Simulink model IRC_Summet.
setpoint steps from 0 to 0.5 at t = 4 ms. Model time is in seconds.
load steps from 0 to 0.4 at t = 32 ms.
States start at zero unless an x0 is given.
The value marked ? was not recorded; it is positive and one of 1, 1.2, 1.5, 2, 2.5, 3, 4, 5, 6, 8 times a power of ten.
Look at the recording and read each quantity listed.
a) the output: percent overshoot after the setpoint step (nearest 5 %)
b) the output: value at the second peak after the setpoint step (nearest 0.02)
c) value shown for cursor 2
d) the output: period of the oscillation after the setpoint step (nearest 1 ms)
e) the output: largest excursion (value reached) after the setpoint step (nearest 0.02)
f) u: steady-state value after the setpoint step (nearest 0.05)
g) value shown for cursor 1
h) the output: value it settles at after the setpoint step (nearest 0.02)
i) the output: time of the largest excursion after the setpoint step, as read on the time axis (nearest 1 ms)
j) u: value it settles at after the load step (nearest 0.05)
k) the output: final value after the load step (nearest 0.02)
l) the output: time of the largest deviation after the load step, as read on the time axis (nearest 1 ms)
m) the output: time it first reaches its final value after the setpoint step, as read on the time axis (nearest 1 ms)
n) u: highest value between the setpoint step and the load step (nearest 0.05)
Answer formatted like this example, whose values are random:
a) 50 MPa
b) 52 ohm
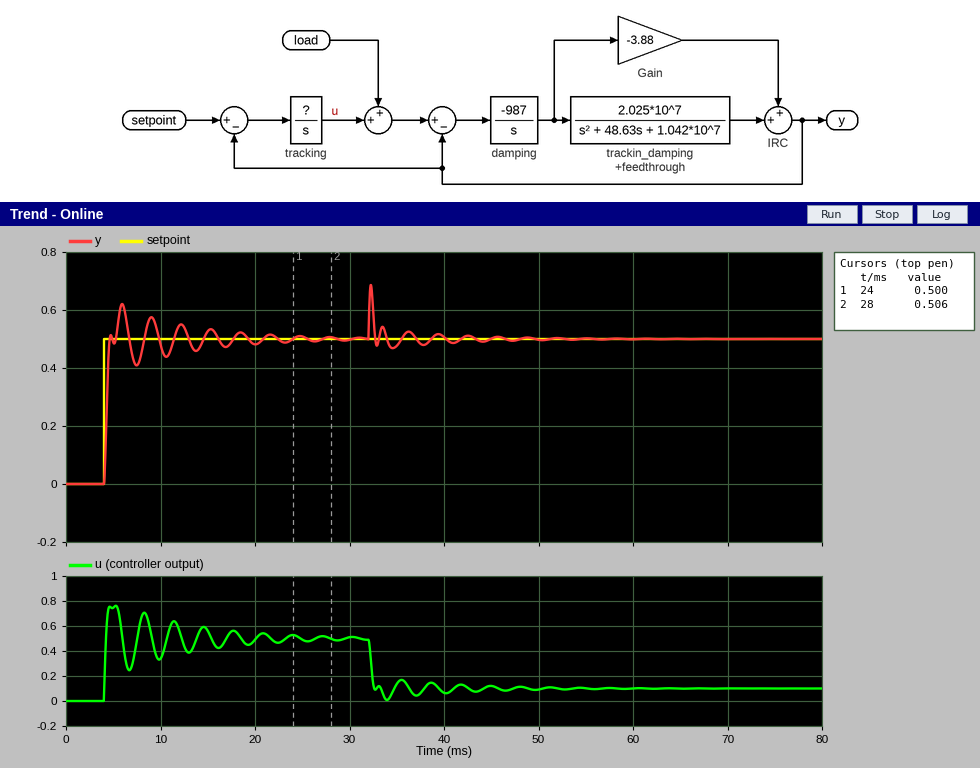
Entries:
a) 25 %
b) 0.58
c) 0.506
d) 3 ms
e) 0.62
f) 0.50
g) 0.500
h) 0.50
i) 6 ms
j) 0.10
k) 0.50
l) 32 ms
m) 5 ms
n) 0.75
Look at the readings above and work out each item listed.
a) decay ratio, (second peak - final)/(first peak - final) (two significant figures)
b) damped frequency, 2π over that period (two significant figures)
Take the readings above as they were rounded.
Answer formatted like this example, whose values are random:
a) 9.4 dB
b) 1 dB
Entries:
a) 0.67
b) 2.1 rad/ms
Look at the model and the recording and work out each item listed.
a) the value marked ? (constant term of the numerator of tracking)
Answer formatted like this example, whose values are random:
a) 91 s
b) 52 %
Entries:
a) 5000
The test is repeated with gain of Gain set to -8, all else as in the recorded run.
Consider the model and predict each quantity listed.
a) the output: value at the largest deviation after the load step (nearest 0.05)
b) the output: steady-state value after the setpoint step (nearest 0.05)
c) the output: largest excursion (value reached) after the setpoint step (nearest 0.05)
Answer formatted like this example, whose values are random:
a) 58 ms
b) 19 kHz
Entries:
a) 0.75
b) 0.50
c) 0.55
